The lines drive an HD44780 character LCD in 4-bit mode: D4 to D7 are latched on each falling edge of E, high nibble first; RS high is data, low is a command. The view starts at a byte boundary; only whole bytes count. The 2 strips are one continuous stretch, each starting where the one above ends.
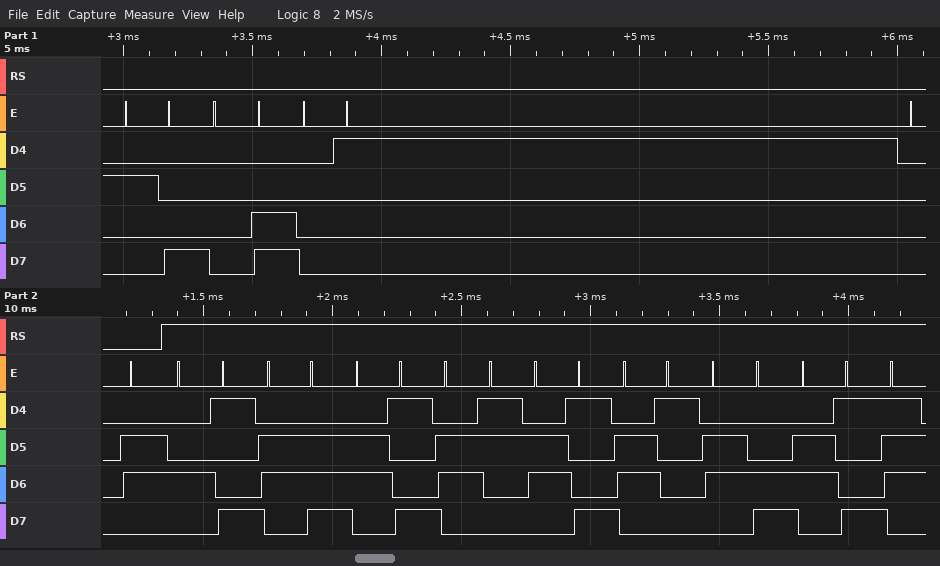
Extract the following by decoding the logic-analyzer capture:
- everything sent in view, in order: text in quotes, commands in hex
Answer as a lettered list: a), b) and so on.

a) 0x28 0x0C 0x01 0x06 "Iniciali"
